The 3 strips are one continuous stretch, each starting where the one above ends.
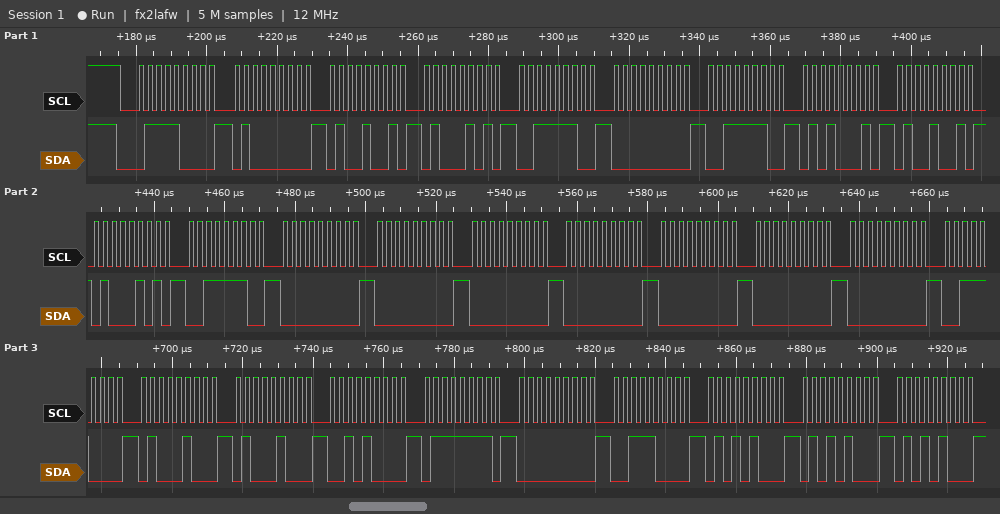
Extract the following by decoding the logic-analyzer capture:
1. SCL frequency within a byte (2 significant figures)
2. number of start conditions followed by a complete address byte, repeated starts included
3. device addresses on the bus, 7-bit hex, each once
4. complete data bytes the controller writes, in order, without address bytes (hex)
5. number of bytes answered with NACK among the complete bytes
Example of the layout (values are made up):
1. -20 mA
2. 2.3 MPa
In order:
1. 400 kHz
2. 1
3. 0x3C
4. 40 49 45 3E 00 3E 51 49 45 3E 00 00 00 00 00 00 00 38 44 44 28 7F 00 38 54 54 54
5. 0
